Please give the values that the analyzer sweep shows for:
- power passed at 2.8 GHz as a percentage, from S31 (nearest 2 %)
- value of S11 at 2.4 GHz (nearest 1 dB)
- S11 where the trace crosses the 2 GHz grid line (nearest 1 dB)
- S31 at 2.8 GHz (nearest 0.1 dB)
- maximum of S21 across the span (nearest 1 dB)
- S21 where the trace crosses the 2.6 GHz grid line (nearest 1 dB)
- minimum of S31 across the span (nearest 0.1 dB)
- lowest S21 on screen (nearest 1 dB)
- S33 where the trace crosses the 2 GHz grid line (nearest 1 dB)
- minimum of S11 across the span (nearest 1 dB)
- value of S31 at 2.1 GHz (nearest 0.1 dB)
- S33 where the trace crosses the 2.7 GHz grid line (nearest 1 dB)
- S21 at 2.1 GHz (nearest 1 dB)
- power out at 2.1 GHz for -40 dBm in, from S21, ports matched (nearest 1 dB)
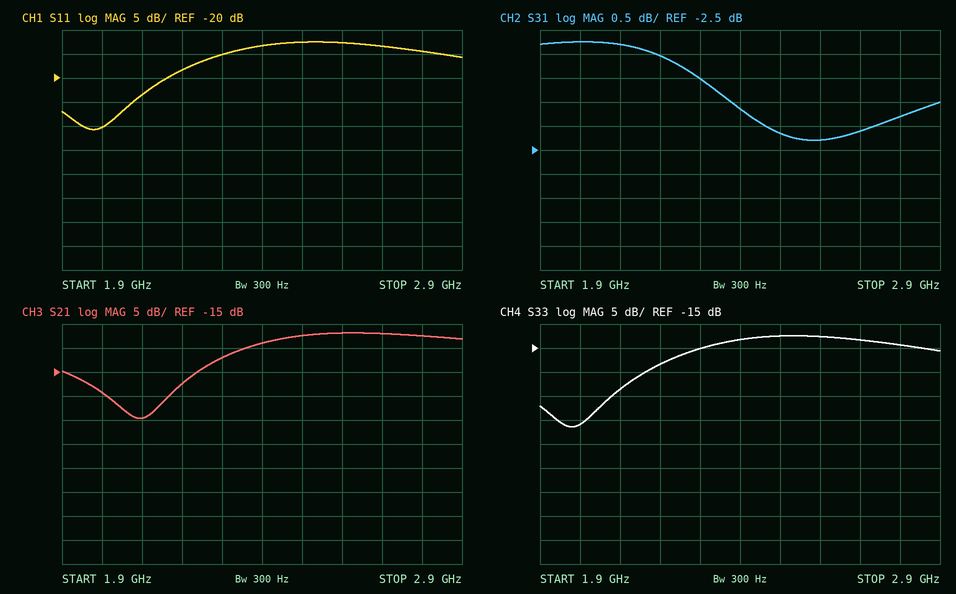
66 %
-13 dB
-30 dB
-1.8 dB
-7 dB
-7 dB
-2.3 dB
-25 dB
-31 dB
-31 dB
-0.3 dB
-13 dB
-25 dB
-65 dBm
